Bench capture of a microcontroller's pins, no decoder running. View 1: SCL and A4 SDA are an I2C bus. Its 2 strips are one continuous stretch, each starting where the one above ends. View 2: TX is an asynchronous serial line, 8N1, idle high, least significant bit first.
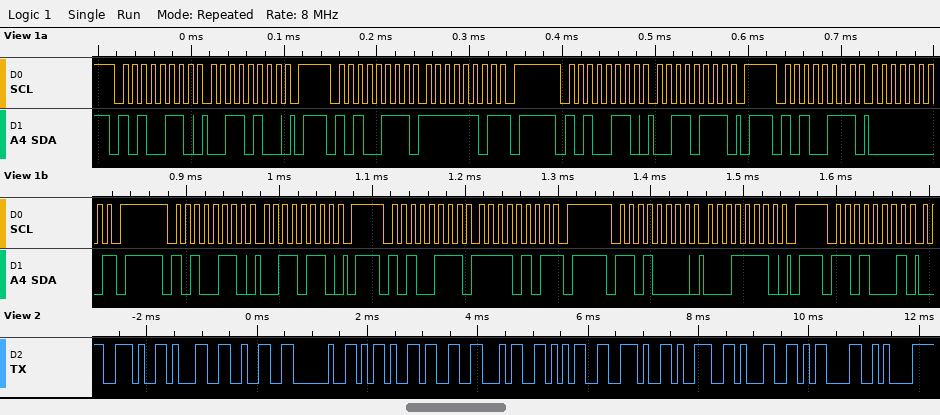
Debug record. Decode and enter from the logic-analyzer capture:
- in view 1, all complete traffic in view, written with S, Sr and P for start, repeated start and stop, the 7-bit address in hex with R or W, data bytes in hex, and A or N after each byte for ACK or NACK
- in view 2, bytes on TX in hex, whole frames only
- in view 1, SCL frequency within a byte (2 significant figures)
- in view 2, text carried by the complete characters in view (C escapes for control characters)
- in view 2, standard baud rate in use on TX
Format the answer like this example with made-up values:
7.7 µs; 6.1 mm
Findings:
S 53W A 34 A P S 53R A FD N P S 53W A 37 A P S 53R A 00 N P S 53W A 36 A P S 53R A F5 N P S 68W A 1E A P S 68R A; 2E 31 32 20 2D 33 34 35 2E 39 31 0D 0A; 100 kHz; ".12 -345.91\r\n"; 9600 baud
